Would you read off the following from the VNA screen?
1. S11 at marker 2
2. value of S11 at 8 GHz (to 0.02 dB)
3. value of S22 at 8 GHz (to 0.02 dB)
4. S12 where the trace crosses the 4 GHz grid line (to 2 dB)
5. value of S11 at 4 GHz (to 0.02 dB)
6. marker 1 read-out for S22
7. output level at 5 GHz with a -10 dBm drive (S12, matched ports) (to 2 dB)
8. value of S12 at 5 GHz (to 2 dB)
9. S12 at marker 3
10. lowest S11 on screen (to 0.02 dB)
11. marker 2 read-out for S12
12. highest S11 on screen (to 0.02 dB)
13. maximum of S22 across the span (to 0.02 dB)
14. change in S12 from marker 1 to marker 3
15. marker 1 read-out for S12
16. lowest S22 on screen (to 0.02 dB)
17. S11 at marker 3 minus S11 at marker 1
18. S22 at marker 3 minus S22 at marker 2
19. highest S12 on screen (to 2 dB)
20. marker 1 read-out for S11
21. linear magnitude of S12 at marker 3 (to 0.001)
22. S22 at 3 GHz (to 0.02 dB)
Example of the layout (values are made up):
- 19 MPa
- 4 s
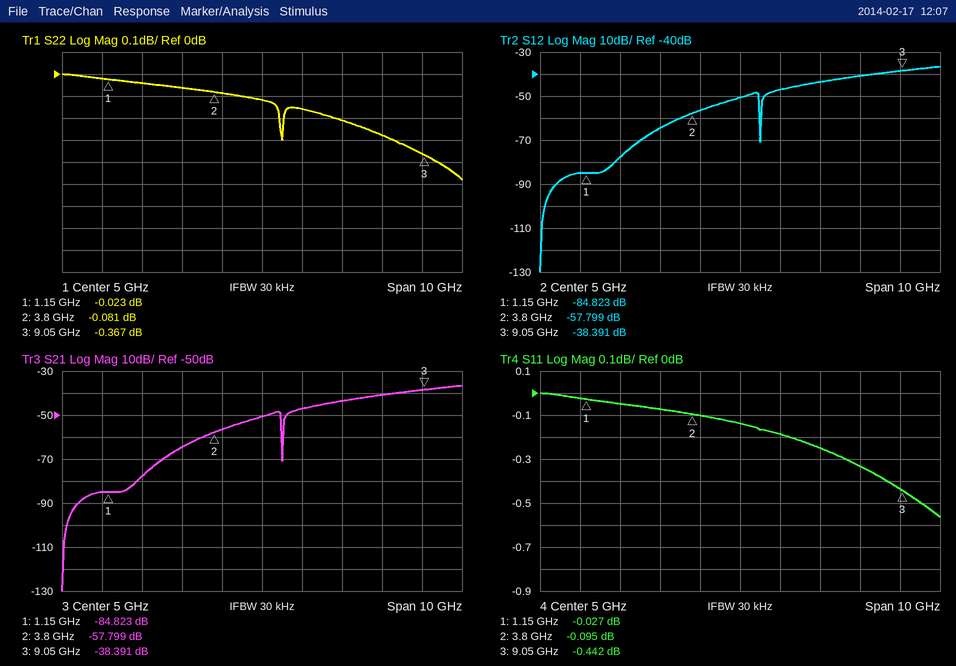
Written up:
- -0.095 dB
- -0.34 dB
- -0.28 dB
- -56 dB
- -0.10 dB
- -0.023 dB
- -60 dBm
- -50 dB
- -38.391 dB
- -0.56 dB
- -57.799 dB
- 0.00 dB
- 0.00 dB
- 46.432 dB
- -84.823 dB
- -0.48 dB
- -0.415 dB
- -0.286 dB
- -36 dB
- -0.027 dB
- 0.012
- -0.06 dB
